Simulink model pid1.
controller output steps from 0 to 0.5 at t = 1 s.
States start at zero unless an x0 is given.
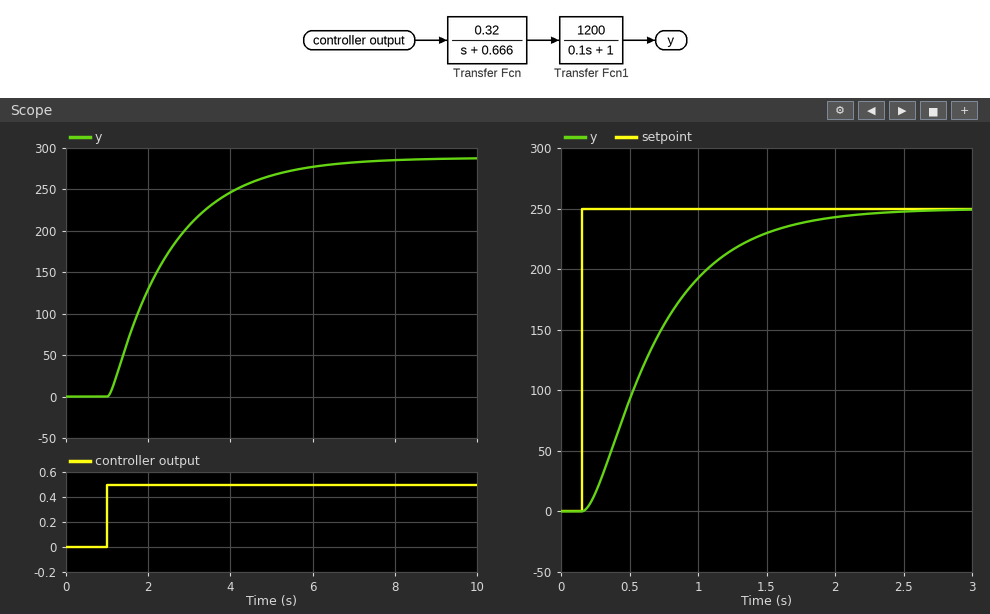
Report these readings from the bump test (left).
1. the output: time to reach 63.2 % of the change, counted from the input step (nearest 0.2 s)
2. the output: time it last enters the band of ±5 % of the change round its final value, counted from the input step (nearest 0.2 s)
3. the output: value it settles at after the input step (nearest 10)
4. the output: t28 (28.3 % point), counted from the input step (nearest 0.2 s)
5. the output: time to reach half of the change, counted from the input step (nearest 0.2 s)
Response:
1.6 s
4.6 s
290
0.6 s
1.2 s
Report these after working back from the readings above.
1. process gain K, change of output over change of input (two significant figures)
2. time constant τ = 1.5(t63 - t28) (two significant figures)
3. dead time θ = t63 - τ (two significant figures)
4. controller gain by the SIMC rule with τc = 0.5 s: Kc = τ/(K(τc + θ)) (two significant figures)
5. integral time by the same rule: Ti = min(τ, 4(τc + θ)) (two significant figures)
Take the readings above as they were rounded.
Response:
580
1.5 s
0.10 s
0.0043
1.5 s
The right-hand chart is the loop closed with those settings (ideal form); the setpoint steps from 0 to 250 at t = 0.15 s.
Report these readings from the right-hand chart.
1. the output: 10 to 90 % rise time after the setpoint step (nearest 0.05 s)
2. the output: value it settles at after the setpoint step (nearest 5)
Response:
1.10 s
250
